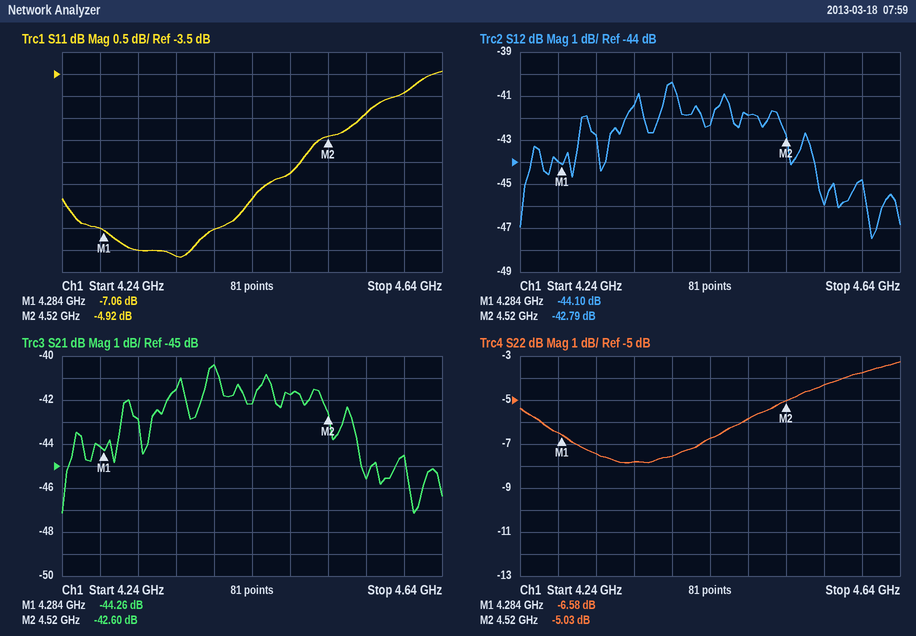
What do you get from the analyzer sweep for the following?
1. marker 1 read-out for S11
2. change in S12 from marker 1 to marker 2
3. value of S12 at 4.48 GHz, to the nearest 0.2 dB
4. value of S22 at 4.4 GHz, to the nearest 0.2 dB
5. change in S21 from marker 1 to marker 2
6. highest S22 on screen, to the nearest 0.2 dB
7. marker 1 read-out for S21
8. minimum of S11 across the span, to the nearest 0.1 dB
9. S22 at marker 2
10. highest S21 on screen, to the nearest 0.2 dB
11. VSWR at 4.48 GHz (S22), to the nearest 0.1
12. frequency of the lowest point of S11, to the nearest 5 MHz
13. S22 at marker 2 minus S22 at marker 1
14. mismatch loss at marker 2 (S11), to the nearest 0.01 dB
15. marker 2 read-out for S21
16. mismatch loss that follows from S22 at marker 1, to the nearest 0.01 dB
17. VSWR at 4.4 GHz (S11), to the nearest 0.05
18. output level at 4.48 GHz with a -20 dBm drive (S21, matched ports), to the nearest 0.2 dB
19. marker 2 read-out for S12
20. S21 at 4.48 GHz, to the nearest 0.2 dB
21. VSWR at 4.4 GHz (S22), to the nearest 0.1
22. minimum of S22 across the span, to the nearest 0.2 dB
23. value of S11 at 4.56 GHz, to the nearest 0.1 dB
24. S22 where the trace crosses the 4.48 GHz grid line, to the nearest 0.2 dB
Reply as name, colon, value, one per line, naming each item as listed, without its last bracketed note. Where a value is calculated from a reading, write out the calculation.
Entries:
marker 1 read-out for S11: -7.06 dB
change in S12 from marker 1 to marker 2: -42.79 − (-44.1) = 1.31 dB
value of S12 at 4.48 GHz, to the nearest 0.2 dB: -41.8 dB
value of S22 at 4.4 GHz, to the nearest 0.2 dB: -7.6 dB
change in S21 from marker 1 to marker 2: -42.6 − (-44.26) = 1.66 dB
highest S22 on screen, to the nearest 0.2 dB: -3.2 dB
marker 1 read-out for S21: -44.26 dB
minimum of S11 across the span, to the nearest 0.1 dB: -7.7 dB
S22 at marker 2: -5.03 dB
highest S21 on screen, to the nearest 0.2 dB: -40.4 dB
VSWR at 4.48 GHz (S22), to the nearest 0.1: |Γ| = 10^(-5.8/20) = 0.5129; VSWR = (1 + 0.5129)/(1 − 0.5129) ≈ 3.1
frequency of the lowest point of S11, to the nearest 5 MHz: 4.365 GHz
S22 at marker 2 minus S22 at marker 1: -5.03 − (-6.58) = 1.55 dB
mismatch loss at marker 2 (S11), to the nearest 0.01 dB: −10 log10(1 − 10^(-4.92/10)) ≈ 1.69 dB
marker 2 read-out for S21: -42.60 dB
mismatch loss that follows from S22 at marker 1, to the nearest 0.01 dB: −10 log10(1 − 10^(-6.58/10)) ≈ 1.08 dB
VSWR at 4.4 GHz (S11), to the nearest 0.05: |Γ| = 10^(-7/20) = 0.4467; VSWR = (1 + 0.4467)/(1 − 0.4467) ≈ 2.61, so 2.60 to the nearest 0.05
output level at 4.48 GHz with a -20 dBm drive (S21, matched ports), to the nearest 0.2 dB: -20 dBm + (-41.8 dB) = -61.8 dBm
marker 2 read-out for S12: -42.79 dB
S21 at 4.48 GHz, to the nearest 0.2 dB: -41.8 dB
VSWR at 4.4 GHz (S22), to the nearest 0.1: |Γ| = 10^(-7.6/20) = 0.4169; VSWR = (1 + 0.4169)/(1 − 0.4169) ≈ 2.4
minimum of S22 across the span, to the nearest 0.2 dB: -7.8 dB
value of S11 at 4.56 GHz, to the nearest 0.1 dB: -4.4 dB
S22 where the trace crosses the 4.48 GHz grid line, to the nearest 0.2 dB: -5.8 dB
